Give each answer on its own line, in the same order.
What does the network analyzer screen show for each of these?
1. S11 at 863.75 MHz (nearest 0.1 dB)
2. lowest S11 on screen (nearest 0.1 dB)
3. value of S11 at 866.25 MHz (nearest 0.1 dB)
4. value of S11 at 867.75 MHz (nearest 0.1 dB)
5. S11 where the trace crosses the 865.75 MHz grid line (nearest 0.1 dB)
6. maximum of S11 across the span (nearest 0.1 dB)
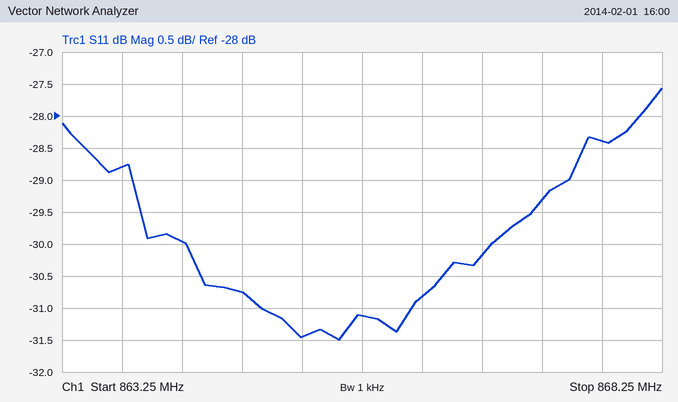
-28.8 dB
-31.5 dB
-30.8 dB
-28.4 dB
-31.1 dB
-27.6 dB
